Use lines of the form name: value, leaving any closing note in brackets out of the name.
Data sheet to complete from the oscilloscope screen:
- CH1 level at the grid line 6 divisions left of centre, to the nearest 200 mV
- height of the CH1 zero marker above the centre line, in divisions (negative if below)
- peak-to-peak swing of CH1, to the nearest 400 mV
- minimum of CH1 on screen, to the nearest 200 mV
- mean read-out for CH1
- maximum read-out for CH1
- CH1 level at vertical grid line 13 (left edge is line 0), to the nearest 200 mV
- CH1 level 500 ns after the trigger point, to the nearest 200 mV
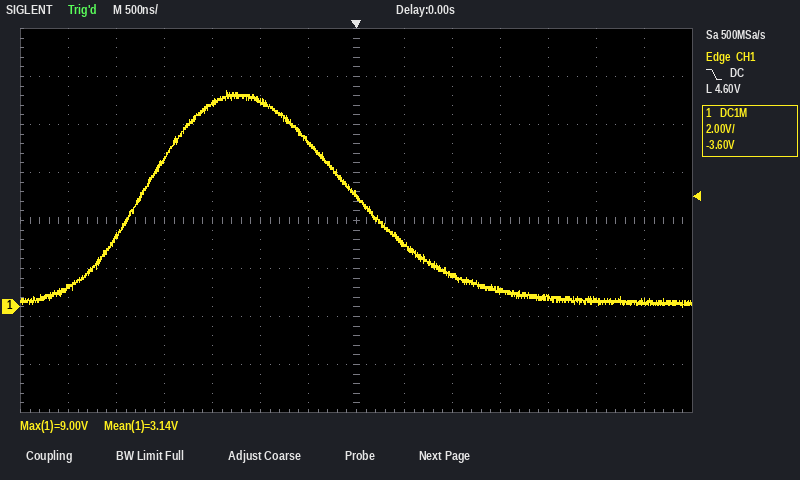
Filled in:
CH1 level at the grid line 6 divisions left of centre, to the nearest 200 mV: 800 mV
height of the CH1 zero marker above the centre line, in divisions: -1.8 div
peak-to-peak swing of CH1, to the nearest 400 mV: 9.2 V
minimum of CH1 on screen, to the nearest 200 mV: 0.0 V
mean read-out for CH1: 3.14 V
maximum read-out for CH1: 9.00 V
CH1 level at vertical grid line 13 (left edge is line 0), to the nearest 200 mV: 200 mV
CH1 level 500 ns after the trigger point, to the nearest 200 mV: 2.6 V
